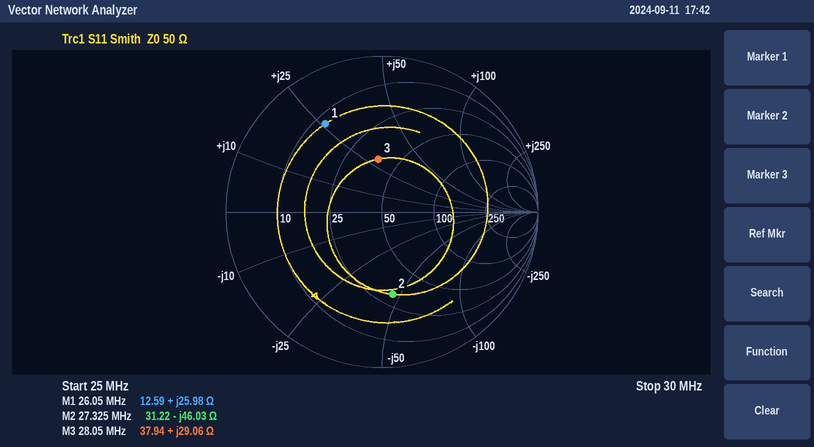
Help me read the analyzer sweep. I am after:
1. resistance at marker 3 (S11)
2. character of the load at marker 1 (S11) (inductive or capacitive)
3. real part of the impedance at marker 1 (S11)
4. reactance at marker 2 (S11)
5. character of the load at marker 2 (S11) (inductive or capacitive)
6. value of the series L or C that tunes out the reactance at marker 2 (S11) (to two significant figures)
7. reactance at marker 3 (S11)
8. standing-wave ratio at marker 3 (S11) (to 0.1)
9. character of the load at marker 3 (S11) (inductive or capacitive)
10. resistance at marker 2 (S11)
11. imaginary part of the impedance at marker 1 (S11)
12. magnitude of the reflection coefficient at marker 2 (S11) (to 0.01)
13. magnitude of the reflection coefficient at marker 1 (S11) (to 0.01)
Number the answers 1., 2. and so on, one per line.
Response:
1. 37.94 Ω
2. inductive
3. 12.59 Ω
4. -46.03 Ω
5. capacitive
6. 270 nH
7. +29.06 Ω
8. 2.0
9. inductive
10. 31.22 Ω
11. +25.98 Ω
12. 0.53
13. 0.67
